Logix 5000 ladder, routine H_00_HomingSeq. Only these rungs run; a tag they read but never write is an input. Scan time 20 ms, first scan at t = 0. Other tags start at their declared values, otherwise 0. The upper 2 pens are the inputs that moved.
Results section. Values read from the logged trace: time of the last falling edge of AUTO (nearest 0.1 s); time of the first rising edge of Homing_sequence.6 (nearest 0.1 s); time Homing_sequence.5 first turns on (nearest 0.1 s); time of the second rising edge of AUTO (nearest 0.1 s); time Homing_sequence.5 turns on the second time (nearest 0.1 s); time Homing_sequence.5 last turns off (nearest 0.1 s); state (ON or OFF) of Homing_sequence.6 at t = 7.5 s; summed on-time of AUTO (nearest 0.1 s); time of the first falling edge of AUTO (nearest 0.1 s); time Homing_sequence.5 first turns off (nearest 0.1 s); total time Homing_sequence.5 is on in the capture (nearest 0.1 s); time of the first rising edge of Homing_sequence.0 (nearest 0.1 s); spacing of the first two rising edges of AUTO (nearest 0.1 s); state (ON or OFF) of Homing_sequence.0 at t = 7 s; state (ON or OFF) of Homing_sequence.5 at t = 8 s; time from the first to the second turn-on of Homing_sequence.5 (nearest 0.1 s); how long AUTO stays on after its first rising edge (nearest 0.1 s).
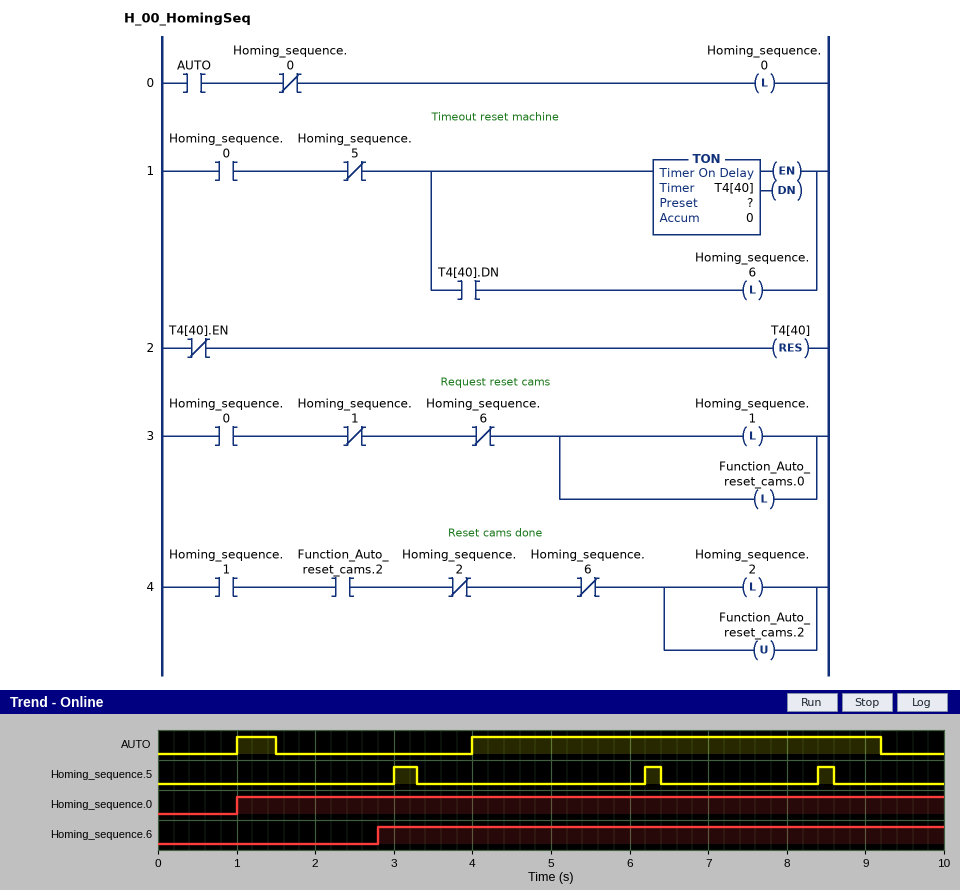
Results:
9.2 s
2.8 s
3.0 s
4.0 s
6.2 s
8.6 s
ON
5.7 s
1.5 s
3.3 s
0.7 s
1.0 s
3.0 s
ON
OFF
3.2 s
0.5 s
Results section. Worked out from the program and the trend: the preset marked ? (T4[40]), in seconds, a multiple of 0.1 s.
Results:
1.8 s
